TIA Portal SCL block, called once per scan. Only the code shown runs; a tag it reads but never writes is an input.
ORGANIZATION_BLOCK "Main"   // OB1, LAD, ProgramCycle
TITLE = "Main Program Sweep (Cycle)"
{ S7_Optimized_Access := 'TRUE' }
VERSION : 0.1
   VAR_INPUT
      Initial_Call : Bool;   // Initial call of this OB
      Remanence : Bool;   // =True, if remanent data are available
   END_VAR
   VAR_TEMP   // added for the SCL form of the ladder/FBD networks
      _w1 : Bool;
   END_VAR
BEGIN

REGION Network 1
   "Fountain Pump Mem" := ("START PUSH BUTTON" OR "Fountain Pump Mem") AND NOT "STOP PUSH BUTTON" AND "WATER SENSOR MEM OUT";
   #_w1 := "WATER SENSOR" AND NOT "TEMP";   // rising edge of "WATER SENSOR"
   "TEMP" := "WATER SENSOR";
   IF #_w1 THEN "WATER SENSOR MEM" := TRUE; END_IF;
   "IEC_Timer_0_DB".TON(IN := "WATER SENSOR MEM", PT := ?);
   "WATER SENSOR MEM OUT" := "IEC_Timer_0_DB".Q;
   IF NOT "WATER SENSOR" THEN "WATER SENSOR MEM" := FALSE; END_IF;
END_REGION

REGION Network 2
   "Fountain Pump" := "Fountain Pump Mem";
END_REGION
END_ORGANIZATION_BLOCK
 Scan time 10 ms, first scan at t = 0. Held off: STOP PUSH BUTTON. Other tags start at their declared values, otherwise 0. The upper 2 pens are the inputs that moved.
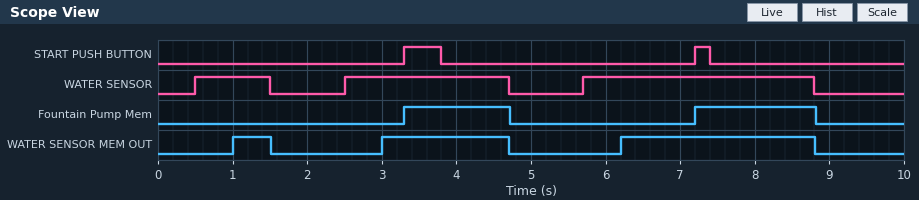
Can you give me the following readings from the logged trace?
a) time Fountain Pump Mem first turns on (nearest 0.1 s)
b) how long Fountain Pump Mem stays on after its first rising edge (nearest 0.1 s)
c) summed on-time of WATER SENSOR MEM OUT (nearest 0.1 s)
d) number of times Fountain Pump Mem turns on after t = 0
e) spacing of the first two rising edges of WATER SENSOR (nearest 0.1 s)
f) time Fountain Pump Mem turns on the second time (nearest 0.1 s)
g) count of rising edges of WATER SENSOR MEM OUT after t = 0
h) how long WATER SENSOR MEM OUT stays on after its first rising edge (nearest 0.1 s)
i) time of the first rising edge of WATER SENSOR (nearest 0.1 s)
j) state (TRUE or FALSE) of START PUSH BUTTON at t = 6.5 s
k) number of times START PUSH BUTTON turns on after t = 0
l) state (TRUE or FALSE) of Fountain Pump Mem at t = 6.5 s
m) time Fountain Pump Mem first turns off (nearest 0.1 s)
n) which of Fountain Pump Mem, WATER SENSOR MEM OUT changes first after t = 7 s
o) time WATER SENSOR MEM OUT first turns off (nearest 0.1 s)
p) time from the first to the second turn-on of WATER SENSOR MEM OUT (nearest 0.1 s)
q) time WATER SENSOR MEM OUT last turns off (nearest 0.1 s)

3.3 s
1.4 s
4.8 s
2
2.0 s
7.2 s
3
0.5 s
0.5 s
FALSE
2
FALSE
4.7 s
Fountain Pump Mem
1.5 s
2.0 s
8.8 s
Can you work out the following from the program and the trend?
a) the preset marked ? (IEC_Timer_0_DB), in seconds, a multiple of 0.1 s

0.5 s
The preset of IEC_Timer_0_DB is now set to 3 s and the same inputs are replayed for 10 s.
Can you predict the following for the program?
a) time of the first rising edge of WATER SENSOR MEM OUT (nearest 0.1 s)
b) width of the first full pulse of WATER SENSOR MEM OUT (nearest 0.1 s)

8.7 s
0.1 s
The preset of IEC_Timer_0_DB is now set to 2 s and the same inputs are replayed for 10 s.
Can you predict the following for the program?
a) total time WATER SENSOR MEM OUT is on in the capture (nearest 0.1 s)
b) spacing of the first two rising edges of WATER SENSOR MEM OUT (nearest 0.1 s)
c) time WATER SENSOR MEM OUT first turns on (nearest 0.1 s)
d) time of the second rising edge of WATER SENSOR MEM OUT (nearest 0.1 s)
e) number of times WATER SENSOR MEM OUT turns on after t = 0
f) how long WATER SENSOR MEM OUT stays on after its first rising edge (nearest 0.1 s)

1.3 s
3.2 s
4.5 s
7.7 s
2
0.2 s
